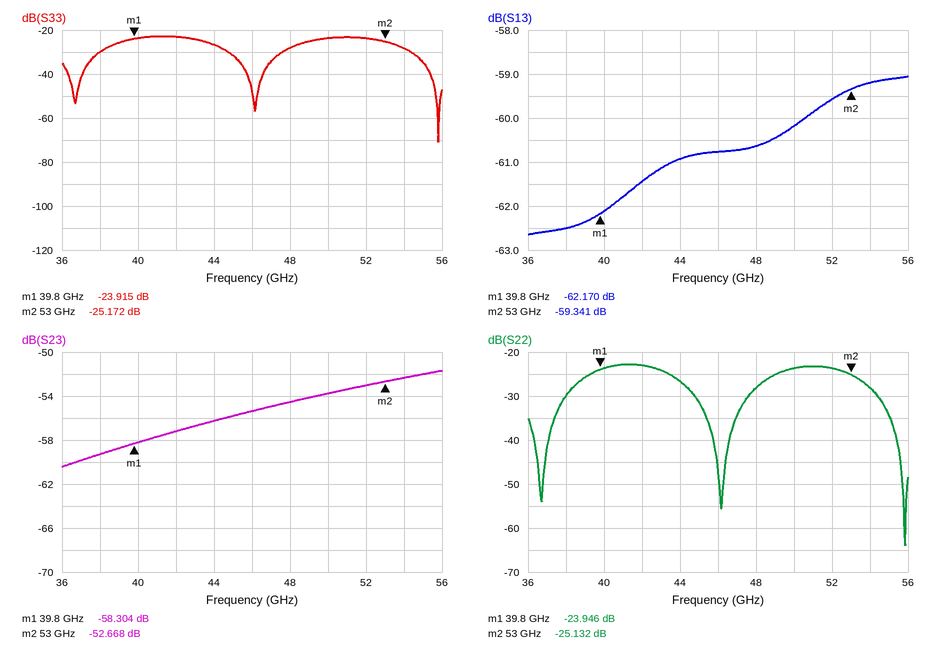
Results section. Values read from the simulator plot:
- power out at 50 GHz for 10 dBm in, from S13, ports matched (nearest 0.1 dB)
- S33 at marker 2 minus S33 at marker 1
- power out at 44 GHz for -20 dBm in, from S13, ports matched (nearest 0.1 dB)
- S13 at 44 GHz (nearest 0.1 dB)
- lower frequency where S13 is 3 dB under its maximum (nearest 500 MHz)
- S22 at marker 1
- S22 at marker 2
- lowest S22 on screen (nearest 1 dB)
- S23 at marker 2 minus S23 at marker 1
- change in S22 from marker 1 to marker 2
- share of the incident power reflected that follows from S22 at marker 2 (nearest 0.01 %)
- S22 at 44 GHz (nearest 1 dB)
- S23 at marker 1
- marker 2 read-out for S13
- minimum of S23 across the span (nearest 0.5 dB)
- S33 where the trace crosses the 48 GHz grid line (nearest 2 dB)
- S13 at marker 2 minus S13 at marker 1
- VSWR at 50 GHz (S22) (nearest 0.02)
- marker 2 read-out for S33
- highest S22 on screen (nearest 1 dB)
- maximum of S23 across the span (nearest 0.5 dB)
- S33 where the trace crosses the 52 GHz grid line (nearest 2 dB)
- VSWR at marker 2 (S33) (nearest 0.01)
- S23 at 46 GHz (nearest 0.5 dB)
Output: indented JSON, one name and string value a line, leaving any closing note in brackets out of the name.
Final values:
{
  "power out at 50 GHz for 10 dBm in, from S13, ports matched": "-50.2 dBm",
  "S33 at marker 2 minus S33 at marker 1": "-1.257 dB",
  "power out at 44 GHz for -20 dBm in, from S13, ports matched": "-80.9 dBm",
  "S13 at 44 GHz": "-60.9 dB",
  "lower frequency where S13 is 3 dB under its maximum": "40.0 GHz",
  "S22 at marker 1": "-23.946 dB",
  "S22 at marker 2": "-25.132 dB",
  "lowest S22 on screen": "-64 dB",
  "S23 at marker 2 minus S23 at marker 1": "5.636 dB",
  "change in S22 from marker 1 to marker 2": "-1.186 dB",
  "share of the incident power reflected that follows from S22 at marker 2": "0.31 %",
  "S22 at 44 GHz": "-27 dB",
  "S23 at marker 1": "-58.304 dB",
  "marker 2 read-out for S13": "-59.341 dB",
  "minimum of S23 across the span": "-60.5 dB",
  "S33 where the trace crosses the 48 GHz grid line": "-28 dB",
  "S13 at marker 2 minus S13 at marker 1": "2.829 dB",
  "VSWR at 50 GHz (S22)": "1.14",
  "marker 2 read-out for S33": "-25.172 dB",
  "highest S22 on screen": "-23 dB",
  "maximum of S23 across the span": "-51.5 dB",
  "S33 where the trace crosses the 52 GHz grid line": "-24 dB",
  "VSWR at marker 2 (S33)": "1.12",
  "S23 at 46 GHz": "-55.5 dB"
}
